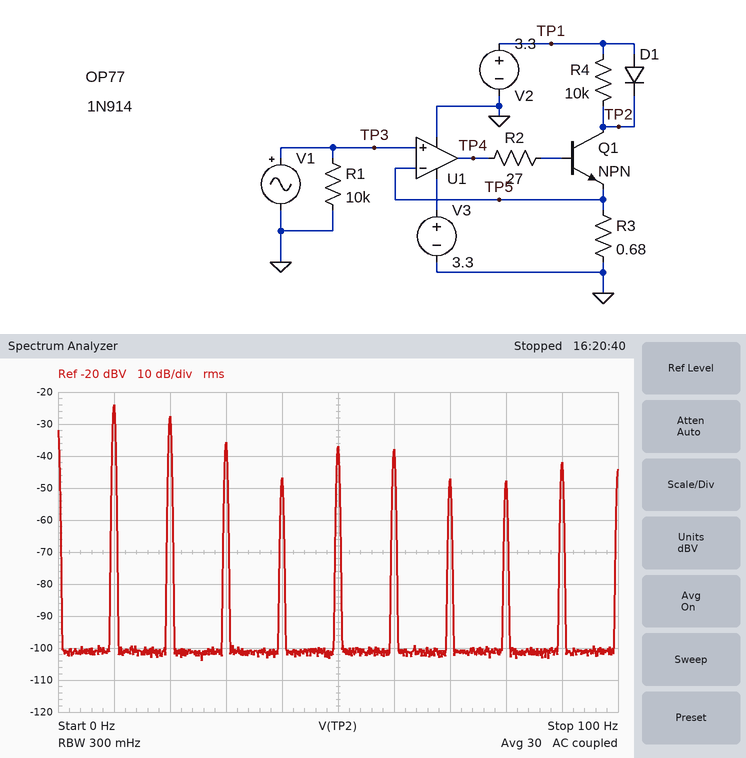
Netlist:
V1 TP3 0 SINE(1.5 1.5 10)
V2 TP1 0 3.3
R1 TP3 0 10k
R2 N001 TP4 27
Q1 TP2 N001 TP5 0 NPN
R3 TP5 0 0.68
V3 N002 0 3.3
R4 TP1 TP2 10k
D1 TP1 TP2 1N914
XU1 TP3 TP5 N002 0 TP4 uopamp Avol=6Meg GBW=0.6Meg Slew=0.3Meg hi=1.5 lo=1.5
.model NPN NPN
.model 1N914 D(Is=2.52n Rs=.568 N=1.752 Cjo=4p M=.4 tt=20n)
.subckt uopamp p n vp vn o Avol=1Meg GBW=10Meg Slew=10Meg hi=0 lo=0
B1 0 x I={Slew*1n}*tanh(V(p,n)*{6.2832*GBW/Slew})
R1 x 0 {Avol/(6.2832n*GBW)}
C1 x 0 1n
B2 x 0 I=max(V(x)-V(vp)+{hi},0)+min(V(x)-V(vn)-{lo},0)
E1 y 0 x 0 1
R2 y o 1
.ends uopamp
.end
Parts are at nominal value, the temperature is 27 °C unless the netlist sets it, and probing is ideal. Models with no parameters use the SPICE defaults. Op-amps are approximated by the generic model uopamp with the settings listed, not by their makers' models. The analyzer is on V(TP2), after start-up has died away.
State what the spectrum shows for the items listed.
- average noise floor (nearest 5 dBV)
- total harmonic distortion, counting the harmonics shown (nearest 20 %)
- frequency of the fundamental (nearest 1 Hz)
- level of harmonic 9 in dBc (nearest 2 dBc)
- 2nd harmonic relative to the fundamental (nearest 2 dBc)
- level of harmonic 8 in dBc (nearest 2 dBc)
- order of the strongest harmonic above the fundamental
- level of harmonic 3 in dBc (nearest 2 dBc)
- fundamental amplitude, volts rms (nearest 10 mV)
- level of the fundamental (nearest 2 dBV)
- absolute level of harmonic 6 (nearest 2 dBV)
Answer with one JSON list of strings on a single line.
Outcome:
["-100 dBV", "80 %", "10 Hz", "-18 dBc", "-4 dBc", "-24 dBc", "2", "-12 dBc", "60 mV", "-24 dBV", "-38 dBV"]
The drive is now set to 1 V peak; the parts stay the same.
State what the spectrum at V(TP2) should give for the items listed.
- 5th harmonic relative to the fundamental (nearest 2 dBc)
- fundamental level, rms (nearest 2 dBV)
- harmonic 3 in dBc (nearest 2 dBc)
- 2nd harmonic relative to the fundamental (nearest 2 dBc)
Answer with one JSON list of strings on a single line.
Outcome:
["-4 dBc", "-38 dBV", "-2 dBc", "0 dBc"]
